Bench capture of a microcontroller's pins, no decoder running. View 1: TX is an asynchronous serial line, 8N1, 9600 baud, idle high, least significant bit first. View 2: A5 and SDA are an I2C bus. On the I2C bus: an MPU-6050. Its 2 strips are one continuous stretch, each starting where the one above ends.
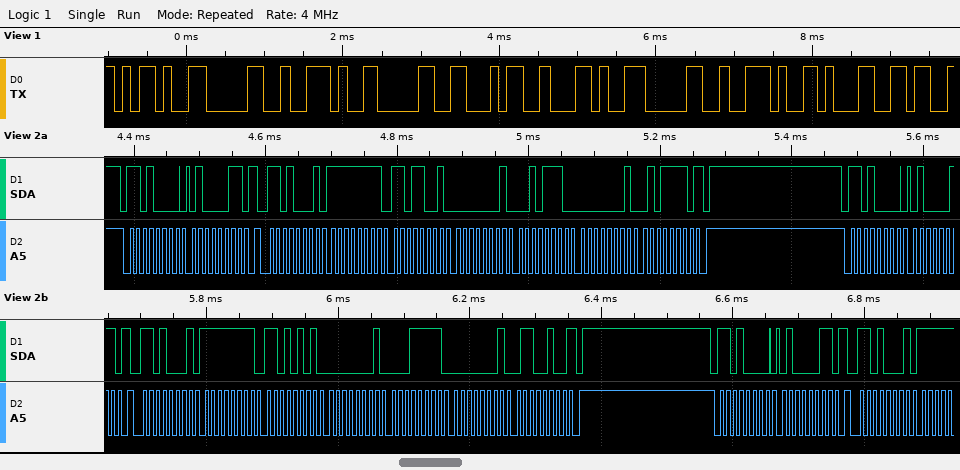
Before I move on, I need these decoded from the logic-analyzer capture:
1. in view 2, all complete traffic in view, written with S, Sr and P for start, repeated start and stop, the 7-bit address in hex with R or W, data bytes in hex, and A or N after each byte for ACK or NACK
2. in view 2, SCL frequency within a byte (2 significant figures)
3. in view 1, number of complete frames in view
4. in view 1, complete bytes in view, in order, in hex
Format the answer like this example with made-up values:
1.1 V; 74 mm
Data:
S 68W A 43 A Sr 68R A FF A D9 A 01 A 2E A 01 A 5E N P S 68W A 43 A Sr 68R A FF A D5 A 01 A 1F A 01 A 64 N P S 68W A 43 A Sr 68R A; 100 kHz; 9; 2D 30 2E 30 34 2C 30 2E 31
